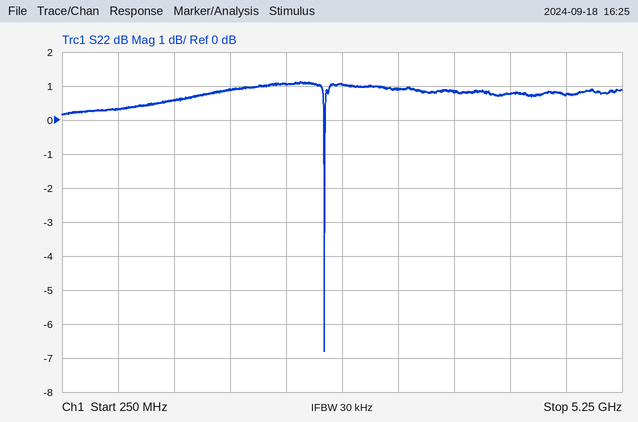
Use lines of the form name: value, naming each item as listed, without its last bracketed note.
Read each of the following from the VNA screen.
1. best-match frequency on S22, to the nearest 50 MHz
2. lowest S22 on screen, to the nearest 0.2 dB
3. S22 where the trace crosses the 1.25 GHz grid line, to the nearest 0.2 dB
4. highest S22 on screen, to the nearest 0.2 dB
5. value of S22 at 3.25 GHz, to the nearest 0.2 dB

best-match frequency on S22, to the nearest 50 MHz: 2.60 GHz
lowest S22 on screen, to the nearest 0.2 dB: -6.8 dB
S22 where the trace crosses the 1.25 GHz grid line, to the nearest 0.2 dB: 0.6 dB
highest S22 on screen, to the nearest 0.2 dB: 1.2 dB
value of S22 at 3.25 GHz, to the nearest 0.2 dB: 1.0 dB
